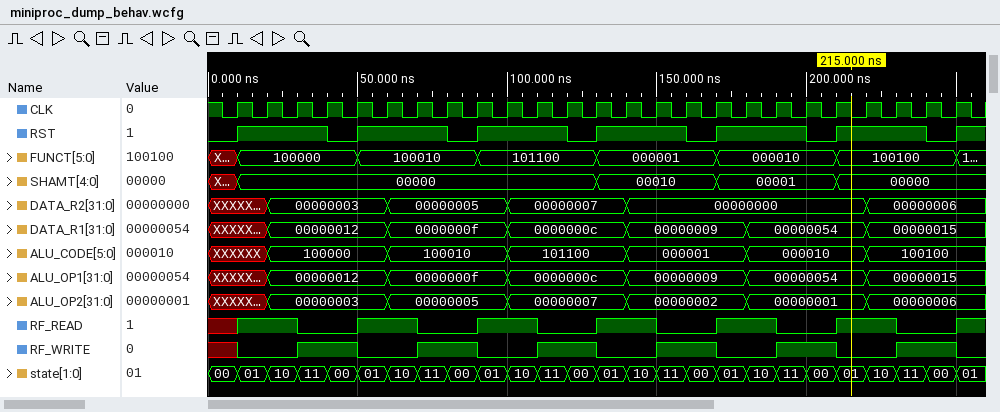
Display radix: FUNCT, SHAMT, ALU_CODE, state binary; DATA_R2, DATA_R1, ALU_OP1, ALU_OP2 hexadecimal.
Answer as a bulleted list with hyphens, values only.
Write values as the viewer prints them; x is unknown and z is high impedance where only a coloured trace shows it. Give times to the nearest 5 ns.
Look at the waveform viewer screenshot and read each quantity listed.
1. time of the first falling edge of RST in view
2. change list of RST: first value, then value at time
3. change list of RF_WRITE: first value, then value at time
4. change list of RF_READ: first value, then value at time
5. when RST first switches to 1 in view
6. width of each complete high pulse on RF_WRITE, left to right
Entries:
- 40 ns
- 0, 1 at 10 ns, 0 at 40 ns, 1 at 50 ns, 0 at 80 ns, 1 at 90 ns, 0 at 120 ns, 1 at 130 ns, 0 at 160 ns, 1 at 170 ns, 0 at 200 ns, 1 at 210 ns, 0 at 240 ns, 1 at 250 ns
- x, 0 at 10 ns, 1 at 30 ns, 0 at 50 ns, 1 at 70 ns, 0 at 90 ns, 1 at 110 ns, 0 at 130 ns, 1 at 150 ns, 0 at 170 ns, 1 at 190 ns, 0 at 210 ns, 1 at 230 ns, 0 at 250 ns
- x, 1 at 10 ns, 0 at 30 ns, 1 at 50 ns, 0 at 70 ns, 1 at 90 ns, 0 at 110 ns, 1 at 130 ns, 0 at 150 ns, 1 at 170 ns, 0 at 190 ns, 1 at 210 ns, 0 at 230 ns, 1 at 250 ns
- 10 ns
- 20 ns, 20 ns, 20 ns, 20 ns, 20 ns, 20 ns
